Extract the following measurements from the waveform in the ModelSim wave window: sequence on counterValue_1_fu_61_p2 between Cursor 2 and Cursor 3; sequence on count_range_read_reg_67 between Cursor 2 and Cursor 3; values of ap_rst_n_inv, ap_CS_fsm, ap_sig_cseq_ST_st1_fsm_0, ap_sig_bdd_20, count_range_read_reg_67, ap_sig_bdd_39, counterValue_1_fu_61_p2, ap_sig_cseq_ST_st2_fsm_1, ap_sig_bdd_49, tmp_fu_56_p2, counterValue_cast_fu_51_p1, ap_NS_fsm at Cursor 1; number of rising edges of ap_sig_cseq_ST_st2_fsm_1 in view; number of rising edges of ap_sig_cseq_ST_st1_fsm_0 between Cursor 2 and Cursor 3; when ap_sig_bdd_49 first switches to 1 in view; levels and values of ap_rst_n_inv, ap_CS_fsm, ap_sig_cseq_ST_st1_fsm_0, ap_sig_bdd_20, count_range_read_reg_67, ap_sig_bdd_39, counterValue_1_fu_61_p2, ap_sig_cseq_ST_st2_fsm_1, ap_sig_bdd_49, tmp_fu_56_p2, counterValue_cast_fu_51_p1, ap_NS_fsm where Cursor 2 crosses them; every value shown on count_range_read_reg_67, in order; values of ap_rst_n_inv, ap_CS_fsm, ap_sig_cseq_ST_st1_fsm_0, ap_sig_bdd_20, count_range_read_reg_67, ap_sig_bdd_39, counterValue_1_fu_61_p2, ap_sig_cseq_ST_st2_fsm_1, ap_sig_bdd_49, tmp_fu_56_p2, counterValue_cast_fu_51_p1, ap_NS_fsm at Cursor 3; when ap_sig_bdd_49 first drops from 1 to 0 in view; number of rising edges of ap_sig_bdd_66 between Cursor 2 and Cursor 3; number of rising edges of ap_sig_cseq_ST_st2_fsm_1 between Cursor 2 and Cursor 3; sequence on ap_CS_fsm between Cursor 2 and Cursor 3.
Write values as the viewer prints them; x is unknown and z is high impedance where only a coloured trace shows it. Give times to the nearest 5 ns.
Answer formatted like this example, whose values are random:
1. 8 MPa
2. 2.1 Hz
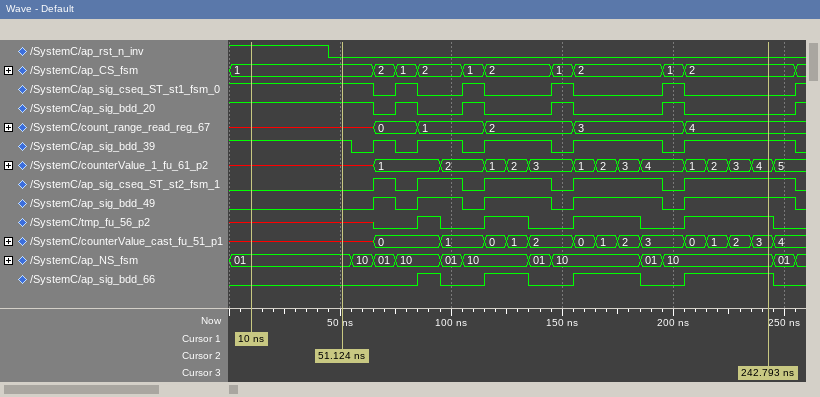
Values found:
1. x, 1, 2, 1, 2, 3, 1, 2, 3, 4, 1, 2, 3, 4
2. x, 0, 1, 2, 3, 4
3. ap_rst_n_inv=1, ap_CS_fsm=1, ap_sig_cseq_ST_st1_fsm_0=1, ap_sig_bdd_20=1, count_range_read_reg_67=x, ap_sig_bdd_39=1, counterValue_1_fu_61_p2=x, ap_sig_cseq_ST_st2_fsm_1=0, ap_sig_bdd_49=0, tmp_fu_56_p2=x, counterValue_cast_fu_51_p1=x, ap_NS_fsm=01
4. 5
5. 4
6. 65 ns
7. ap_rst_n_inv=0, ap_CS_fsm=1, ap_sig_cseq_ST_st1_fsm_0=1, ap_sig_bdd_20=1, count_range_read_reg_67=x, ap_sig_bdd_39=1, counterValue_1_fu_61_p2=x, ap_sig_cseq_ST_st2_fsm_1=0, ap_sig_bdd_49=0, tmp_fu_56_p2=x, counterValue_cast_fu_51_p1=x, ap_NS_fsm=01
8. x, 0, 1, 2, 3, 4
9. ap_rst_n_inv=0, ap_CS_fsm=2, ap_sig_cseq_ST_st1_fsm_0=0, ap_sig_bdd_20=0, count_range_read_reg_67=4, ap_sig_bdd_39=1, counterValue_1_fu_61_p2=4, ap_sig_cseq_ST_st2_fsm_1=1, ap_sig_bdd_49=1, tmp_fu_56_p2=1, counterValue_cast_fu_51_p1=3, ap_NS_fsm=10
10. 75 ns
11. 4
12. 5
13. 1, 2, 1, 2, 1, 2, 1, 2, 1, 2
